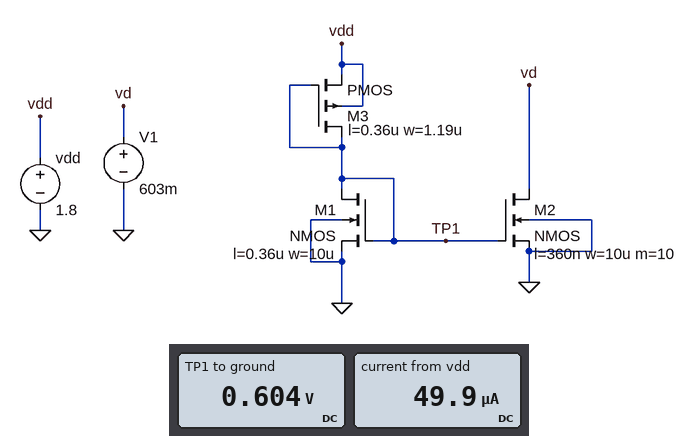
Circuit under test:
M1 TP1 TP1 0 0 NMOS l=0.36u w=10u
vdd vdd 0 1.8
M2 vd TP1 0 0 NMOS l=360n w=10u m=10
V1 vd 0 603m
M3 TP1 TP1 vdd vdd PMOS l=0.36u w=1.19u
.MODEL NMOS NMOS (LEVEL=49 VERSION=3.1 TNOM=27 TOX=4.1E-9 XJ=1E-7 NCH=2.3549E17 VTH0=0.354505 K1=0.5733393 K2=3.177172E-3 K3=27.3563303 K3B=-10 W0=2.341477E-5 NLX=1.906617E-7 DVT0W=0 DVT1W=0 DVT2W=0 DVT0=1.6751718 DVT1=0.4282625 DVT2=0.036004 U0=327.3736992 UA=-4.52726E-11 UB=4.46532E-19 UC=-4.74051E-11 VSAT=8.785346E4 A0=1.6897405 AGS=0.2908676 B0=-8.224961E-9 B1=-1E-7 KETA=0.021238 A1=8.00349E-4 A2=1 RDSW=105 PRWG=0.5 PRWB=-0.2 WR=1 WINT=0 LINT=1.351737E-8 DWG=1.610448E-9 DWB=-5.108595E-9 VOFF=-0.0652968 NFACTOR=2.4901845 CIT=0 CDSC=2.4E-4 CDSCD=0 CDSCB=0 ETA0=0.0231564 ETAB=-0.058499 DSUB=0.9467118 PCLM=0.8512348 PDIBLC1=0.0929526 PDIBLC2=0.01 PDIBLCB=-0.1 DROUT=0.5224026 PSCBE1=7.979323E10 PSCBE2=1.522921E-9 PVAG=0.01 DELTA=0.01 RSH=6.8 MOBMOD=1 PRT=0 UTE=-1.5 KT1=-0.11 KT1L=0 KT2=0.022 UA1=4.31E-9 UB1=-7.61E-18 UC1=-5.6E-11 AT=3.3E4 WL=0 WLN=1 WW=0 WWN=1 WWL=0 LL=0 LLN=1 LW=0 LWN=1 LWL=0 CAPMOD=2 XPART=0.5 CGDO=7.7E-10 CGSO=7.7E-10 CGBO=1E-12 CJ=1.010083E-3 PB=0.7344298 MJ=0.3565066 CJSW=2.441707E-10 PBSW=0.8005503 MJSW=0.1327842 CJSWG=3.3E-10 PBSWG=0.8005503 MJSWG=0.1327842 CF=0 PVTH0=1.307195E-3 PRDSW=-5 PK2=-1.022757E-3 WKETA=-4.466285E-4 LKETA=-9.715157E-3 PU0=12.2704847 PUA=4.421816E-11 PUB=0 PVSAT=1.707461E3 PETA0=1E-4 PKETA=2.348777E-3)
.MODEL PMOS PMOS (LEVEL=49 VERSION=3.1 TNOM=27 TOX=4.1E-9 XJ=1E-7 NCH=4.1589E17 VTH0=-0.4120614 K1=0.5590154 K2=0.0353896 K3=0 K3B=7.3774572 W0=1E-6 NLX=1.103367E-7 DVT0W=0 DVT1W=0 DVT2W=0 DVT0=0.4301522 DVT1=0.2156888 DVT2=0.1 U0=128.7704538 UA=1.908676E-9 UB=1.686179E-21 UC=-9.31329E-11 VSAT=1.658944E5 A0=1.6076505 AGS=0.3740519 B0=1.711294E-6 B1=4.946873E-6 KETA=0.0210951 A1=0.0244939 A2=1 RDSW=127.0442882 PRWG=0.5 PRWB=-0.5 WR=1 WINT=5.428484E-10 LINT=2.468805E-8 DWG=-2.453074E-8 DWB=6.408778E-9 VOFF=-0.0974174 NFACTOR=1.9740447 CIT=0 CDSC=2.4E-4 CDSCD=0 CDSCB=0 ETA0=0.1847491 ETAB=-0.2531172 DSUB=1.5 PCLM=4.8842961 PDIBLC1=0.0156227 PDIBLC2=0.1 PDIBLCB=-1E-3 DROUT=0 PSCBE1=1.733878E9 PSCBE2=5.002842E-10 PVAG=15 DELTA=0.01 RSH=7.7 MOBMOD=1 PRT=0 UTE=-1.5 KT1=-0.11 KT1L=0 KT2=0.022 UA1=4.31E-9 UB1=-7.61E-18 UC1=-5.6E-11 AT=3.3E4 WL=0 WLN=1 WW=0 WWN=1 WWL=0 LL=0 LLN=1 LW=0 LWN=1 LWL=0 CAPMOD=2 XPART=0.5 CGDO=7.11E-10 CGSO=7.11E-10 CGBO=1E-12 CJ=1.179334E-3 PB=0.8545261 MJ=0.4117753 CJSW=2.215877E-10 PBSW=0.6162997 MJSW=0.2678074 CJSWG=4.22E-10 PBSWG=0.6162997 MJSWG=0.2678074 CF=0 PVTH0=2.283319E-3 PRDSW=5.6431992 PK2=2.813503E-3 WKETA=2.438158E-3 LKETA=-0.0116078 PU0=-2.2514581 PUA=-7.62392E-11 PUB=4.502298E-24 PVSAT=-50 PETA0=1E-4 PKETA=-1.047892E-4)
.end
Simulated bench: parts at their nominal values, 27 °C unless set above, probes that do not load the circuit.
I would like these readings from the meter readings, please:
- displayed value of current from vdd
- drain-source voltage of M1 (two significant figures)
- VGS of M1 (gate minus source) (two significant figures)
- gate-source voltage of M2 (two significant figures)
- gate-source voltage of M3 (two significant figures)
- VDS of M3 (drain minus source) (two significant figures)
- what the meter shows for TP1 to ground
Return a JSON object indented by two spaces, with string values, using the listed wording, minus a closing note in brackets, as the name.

{
  "displayed value of current from vdd": "49.9 µA",
  "drain-source voltage of M1": "600 mV",
  "VGS of M1 (gate minus source)": "600 mV",
  "gate-source voltage of M2": "600 mV",
  "gate-source voltage of M3": "-1.2 V",
  "VDS of M3 (drain minus source)": "-1.2 V",
  "what the meter shows for TP1 to ground": "0.604 V"
}
